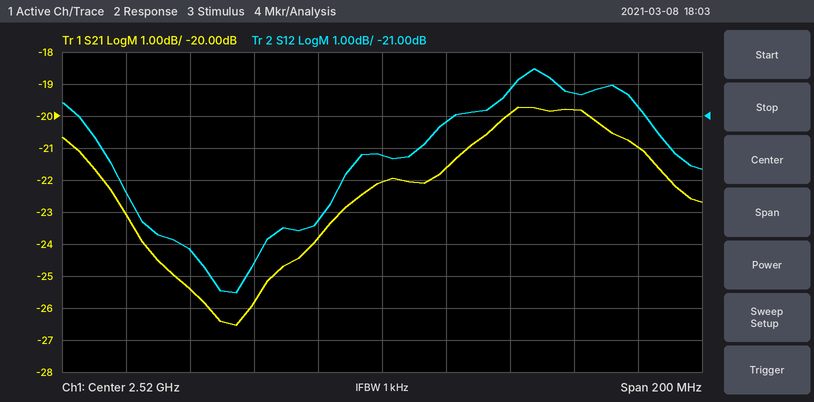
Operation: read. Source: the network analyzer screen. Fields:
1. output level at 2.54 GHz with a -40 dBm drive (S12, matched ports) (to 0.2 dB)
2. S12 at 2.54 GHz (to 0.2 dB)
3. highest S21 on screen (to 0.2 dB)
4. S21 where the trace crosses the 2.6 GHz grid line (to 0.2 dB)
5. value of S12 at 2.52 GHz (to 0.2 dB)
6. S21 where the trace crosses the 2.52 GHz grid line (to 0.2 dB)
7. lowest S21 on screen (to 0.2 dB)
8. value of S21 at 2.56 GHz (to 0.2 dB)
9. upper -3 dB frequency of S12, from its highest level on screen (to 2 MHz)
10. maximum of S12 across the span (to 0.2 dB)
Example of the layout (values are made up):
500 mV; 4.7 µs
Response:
-61.2 dBm; -21.2 dB; -19.8 dB; -21.0 dB; -22.2 dB; -22.0 dB; -26.6 dB; -20.0 dB; 2.616 GHz; -19.6 dB
